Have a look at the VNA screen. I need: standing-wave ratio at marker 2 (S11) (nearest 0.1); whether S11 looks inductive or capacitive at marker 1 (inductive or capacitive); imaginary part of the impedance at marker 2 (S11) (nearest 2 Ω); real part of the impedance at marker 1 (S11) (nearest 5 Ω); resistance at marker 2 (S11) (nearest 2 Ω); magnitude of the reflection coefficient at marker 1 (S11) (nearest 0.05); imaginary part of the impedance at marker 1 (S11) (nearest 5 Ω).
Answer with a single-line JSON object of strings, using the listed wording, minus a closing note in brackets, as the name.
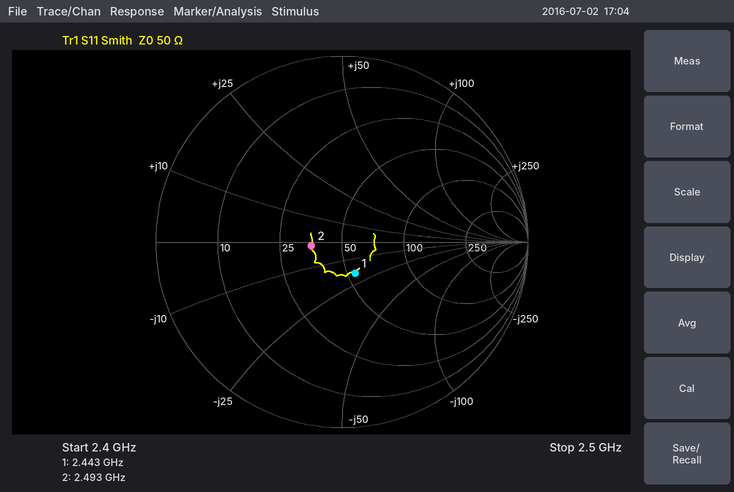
{"standing-wave ratio at marker 2 (S11)": "1.4", "whether S11 looks inductive or capacitive at marker 1": "capacitive", "imaginary part of the impedance at marker 2 (S11)": "-2 Ω", "real part of the impedance at marker 1 (S11)": "55 Ω", "resistance at marker 2 (S11)": "36 Ω", "magnitude of the reflection coefficient at marker 1 (S11)": "0.20", "imaginary part of the impedance at marker 1 (S11)": "-20 Ω"}
